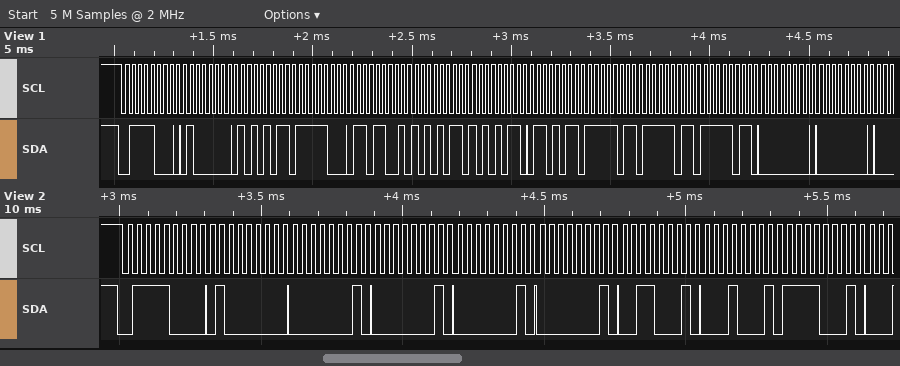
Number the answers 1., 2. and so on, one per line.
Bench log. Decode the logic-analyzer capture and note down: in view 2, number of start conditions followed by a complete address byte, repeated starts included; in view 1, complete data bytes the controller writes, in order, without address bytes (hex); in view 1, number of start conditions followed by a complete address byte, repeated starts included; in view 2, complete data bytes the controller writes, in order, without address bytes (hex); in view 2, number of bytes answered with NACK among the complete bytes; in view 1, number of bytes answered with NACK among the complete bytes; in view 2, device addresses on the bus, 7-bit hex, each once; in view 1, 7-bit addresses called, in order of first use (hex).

1. 1
2. 40 AB F8 D9 AB AB 6B FB FB FB 00 00
3. 1
4. 40 01 01 01 01 31 11 F1
5. 0
6. 0
7. 0x3C
8. 0x3C
